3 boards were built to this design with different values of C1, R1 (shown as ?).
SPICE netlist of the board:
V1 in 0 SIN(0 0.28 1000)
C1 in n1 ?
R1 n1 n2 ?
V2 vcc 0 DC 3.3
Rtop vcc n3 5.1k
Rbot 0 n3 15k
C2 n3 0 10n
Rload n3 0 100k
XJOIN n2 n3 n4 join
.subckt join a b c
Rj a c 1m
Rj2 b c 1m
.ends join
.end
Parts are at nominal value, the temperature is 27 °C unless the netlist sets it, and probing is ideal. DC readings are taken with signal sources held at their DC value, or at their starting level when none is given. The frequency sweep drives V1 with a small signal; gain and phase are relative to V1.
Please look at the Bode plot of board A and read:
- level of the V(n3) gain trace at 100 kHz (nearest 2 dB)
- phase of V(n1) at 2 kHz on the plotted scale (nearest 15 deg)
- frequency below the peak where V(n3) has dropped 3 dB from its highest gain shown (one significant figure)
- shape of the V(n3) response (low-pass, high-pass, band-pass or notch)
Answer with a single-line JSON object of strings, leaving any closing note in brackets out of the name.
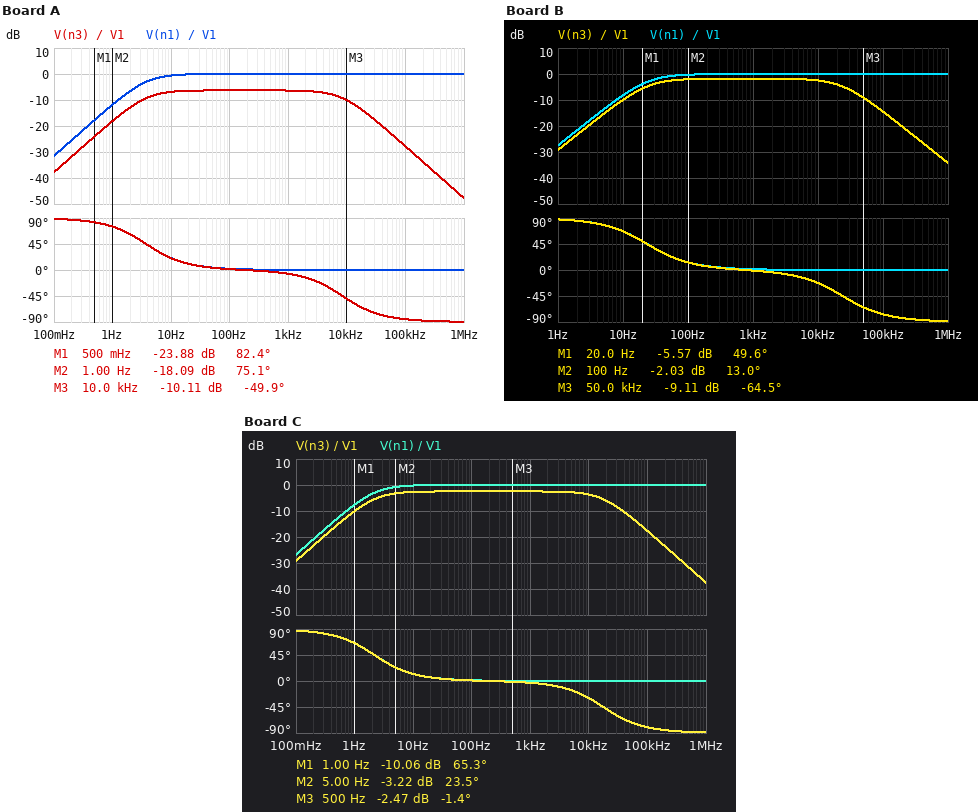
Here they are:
{"level of the V(n3) gain trace at 100 kHz": "-28 dB", "phase of V(n1) at 2 kHz on the plotted scale": "0 deg", "frequency below the peak where V(n3) has dropped 3 dB from its highest gain shown": "4 Hz", "shape of the V(n3) response": "band-pass"}
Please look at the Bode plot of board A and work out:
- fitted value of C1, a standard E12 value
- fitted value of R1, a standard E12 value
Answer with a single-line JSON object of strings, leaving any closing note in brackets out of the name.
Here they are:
{"fitted value of C1, a standard E12 value": "5.6 µF", "fitted value of R1, a standard E12 value": "3.9 kΩ"}
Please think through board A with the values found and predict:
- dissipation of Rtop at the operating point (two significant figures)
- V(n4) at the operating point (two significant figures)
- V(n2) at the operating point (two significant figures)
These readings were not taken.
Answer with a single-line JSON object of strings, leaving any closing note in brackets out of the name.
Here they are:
{"dissipation of Rtop at the operating point": "170 µW", "V(n4) at the operating point": "2.4 V", "V(n2) at the operating point": "2.4 V"}
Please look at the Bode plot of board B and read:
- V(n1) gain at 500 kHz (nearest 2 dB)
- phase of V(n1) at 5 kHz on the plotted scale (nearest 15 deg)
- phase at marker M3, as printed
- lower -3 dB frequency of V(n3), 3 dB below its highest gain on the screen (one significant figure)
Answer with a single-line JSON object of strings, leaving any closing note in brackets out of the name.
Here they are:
{"V(n1) gain at 500 kHz": "0 dB", "phase of V(n1) at 5 kHz on the plotted scale": "0 deg", "phase at marker M3, as printed": "-64.5 deg", "lower -3 dB frequency of V(n3), 3 dB below its highest gain on the screen": "20 Hz"}
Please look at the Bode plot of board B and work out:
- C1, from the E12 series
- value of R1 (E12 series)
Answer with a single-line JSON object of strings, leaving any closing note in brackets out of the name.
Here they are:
{"C1, from the E12 series": "1.5 µF", "value of R1": "820 Ω"}
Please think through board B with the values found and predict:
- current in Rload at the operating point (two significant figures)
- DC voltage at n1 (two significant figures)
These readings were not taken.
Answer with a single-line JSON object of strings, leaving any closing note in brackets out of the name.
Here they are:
{"current in Rload at the operating point": "24 µA", "DC voltage at n1": "2.4 V"}
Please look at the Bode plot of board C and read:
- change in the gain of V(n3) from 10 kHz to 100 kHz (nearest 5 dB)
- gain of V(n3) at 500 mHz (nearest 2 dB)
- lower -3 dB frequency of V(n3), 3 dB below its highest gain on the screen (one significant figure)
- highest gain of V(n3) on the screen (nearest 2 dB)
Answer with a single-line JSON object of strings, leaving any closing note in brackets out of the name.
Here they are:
{"change in the gain of V(n3) from 10 kHz to 100 kHz": "-15 dB", "gain of V(n3) at 500 mHz": "-16 dB", "lower -3 dB frequency of V(n3), 3 dB below its highest gain on the screen": "2 Hz", "highest gain of V(n3) on the screen": "-2 dB"}
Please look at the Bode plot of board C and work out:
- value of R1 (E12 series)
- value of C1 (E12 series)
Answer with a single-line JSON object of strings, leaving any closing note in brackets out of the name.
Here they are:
{"value of R1": "1.2 kΩ", "value of C1": "15 µF"}
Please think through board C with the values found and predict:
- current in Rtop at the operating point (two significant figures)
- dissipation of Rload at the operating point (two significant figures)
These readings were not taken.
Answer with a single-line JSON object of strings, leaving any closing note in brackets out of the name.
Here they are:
{"current in Rtop at the operating point": "180 µA", "dissipation of Rload at the operating point": "56 µW"}
